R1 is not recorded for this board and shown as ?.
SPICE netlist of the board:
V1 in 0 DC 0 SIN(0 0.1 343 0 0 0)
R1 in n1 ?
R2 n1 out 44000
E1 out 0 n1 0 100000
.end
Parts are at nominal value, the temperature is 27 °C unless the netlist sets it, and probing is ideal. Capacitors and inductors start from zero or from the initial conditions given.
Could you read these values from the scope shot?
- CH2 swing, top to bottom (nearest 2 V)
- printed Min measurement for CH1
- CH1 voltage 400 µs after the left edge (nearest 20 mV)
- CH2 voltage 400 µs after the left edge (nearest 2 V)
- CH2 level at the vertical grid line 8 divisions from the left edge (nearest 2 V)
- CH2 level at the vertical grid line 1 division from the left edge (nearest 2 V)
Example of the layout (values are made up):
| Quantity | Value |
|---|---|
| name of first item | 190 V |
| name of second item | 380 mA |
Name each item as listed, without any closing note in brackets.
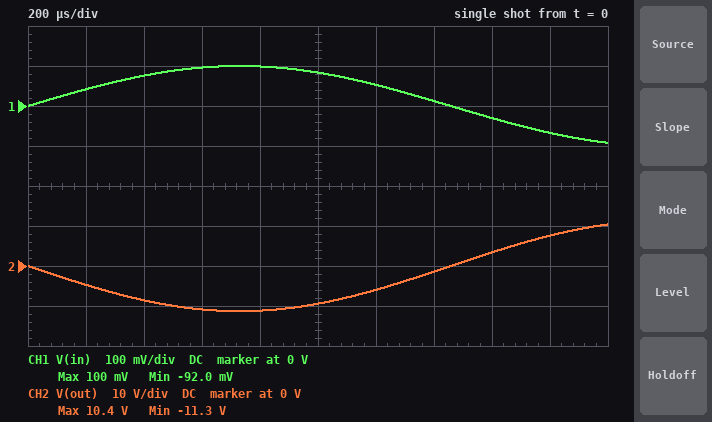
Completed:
| Quantity | Value |
|---|---|
| CH2 swing, top to bottom | 22 V |
| printed Min measurement for CH1 | -92.0 mV |
| CH1 voltage 400 µs after the left edge | 80 mV |
| CH2 voltage 400 µs after the left edge | -8 V |
| CH2 level at the vertical grid line 8 divisions from the left edge | 4 V |
| CH2 level at the vertical grid line 1 division from the left edge | -4 V |
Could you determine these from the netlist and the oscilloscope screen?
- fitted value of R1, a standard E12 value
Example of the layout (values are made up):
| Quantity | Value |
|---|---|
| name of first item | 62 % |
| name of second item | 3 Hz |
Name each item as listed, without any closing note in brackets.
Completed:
| Quantity | Value |
|---|---|
| fitted value of R1, a standard E12 value | 390 Ω |
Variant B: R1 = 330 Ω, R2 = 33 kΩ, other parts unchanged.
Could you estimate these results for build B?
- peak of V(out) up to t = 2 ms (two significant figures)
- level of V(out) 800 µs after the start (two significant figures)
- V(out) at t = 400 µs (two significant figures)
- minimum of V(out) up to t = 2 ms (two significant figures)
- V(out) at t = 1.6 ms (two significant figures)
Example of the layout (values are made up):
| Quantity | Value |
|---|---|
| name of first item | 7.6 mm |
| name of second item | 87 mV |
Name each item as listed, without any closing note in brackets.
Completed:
| Quantity | Value |
|---|---|
| peak of V(out) up to t = 2 ms | 9.2 V |
| level of V(out) 800 µs after the start | -9.9 V |
| V(out) at t = 400 µs | -7.6 V |
| minimum of V(out) up to t = 2 ms | -10 V |
| V(out) at t = 1.6 ms | 3.0 V |
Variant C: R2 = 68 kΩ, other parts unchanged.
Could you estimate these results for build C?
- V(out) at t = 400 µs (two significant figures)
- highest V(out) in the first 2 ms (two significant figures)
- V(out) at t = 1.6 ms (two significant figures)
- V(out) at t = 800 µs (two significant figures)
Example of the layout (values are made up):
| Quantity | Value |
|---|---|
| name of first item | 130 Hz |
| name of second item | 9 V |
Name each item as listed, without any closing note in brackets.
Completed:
| Quantity | Value |
|---|---|
| V(out) at t = 400 µs | -13 V |
| highest V(out) in the first 2 ms | 16 V |
| V(out) at t = 1.6 ms | 5.3 V |
| V(out) at t = 800 µs | -17 V |
